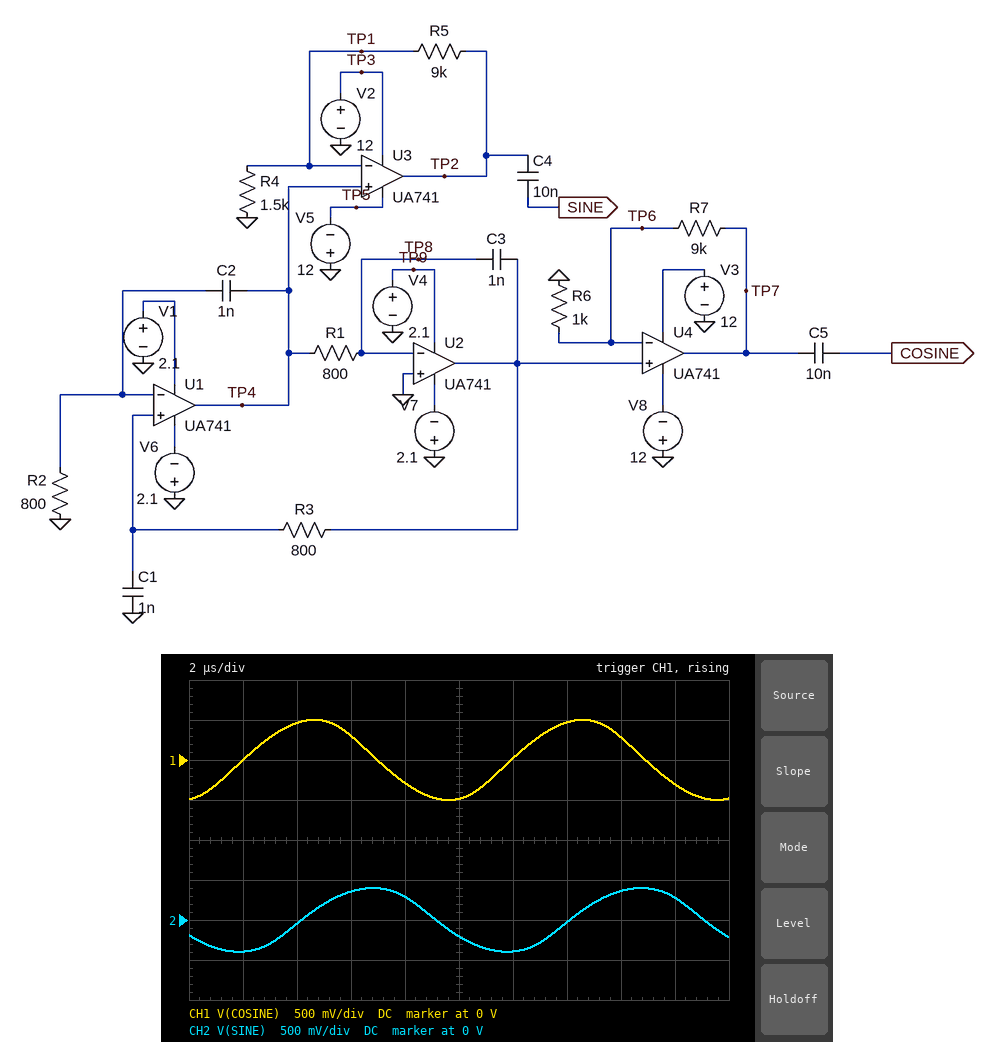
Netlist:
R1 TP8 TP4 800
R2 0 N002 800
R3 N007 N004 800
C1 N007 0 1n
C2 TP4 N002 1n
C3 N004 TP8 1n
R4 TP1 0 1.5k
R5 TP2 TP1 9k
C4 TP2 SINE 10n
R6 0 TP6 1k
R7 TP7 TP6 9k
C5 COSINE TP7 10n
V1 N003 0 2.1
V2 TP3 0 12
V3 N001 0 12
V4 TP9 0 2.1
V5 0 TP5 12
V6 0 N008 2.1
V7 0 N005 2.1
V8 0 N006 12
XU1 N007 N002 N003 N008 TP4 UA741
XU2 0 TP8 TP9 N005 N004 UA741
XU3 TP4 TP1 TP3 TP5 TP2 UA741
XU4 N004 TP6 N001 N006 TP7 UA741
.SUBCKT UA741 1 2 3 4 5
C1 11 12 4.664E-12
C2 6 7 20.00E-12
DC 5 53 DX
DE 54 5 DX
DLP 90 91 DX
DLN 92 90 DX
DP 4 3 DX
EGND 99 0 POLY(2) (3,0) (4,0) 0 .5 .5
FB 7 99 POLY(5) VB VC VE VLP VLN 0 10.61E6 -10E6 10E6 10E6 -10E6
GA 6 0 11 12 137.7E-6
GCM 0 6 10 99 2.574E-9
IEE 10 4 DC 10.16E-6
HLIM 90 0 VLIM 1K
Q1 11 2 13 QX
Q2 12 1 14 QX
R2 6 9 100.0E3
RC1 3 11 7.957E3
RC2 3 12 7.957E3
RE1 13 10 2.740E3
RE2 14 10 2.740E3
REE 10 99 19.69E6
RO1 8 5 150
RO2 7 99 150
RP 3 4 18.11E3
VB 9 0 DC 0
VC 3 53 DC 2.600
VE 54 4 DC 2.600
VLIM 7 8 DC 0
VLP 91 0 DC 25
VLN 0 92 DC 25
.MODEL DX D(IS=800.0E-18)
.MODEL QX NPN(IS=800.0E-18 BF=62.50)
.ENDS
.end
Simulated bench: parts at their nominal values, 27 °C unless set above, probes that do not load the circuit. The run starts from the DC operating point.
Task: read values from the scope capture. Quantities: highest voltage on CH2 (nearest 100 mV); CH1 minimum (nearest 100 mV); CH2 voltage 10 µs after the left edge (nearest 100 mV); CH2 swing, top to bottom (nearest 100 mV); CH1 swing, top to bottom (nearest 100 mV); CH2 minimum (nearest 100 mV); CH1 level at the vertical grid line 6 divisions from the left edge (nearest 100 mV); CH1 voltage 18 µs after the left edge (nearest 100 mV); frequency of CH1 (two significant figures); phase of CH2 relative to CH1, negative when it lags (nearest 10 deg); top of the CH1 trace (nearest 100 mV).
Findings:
400 mV
-500 mV
-200 mV
800 mV
1.0 V
-400 mV
0 V
-300 mV
100 kHz
-80 deg
500 mV
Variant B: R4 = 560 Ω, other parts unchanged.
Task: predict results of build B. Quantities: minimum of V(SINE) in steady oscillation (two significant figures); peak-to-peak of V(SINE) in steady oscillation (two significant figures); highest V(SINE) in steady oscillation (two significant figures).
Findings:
-600 mV
1.2 V
610 mV
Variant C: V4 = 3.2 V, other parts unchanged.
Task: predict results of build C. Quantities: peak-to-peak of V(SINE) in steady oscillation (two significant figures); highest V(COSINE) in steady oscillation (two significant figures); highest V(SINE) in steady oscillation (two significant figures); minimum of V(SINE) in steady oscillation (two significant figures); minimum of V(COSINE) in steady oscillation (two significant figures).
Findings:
970 mV
840 mV
530 mV
-450 mV
-610 mV
